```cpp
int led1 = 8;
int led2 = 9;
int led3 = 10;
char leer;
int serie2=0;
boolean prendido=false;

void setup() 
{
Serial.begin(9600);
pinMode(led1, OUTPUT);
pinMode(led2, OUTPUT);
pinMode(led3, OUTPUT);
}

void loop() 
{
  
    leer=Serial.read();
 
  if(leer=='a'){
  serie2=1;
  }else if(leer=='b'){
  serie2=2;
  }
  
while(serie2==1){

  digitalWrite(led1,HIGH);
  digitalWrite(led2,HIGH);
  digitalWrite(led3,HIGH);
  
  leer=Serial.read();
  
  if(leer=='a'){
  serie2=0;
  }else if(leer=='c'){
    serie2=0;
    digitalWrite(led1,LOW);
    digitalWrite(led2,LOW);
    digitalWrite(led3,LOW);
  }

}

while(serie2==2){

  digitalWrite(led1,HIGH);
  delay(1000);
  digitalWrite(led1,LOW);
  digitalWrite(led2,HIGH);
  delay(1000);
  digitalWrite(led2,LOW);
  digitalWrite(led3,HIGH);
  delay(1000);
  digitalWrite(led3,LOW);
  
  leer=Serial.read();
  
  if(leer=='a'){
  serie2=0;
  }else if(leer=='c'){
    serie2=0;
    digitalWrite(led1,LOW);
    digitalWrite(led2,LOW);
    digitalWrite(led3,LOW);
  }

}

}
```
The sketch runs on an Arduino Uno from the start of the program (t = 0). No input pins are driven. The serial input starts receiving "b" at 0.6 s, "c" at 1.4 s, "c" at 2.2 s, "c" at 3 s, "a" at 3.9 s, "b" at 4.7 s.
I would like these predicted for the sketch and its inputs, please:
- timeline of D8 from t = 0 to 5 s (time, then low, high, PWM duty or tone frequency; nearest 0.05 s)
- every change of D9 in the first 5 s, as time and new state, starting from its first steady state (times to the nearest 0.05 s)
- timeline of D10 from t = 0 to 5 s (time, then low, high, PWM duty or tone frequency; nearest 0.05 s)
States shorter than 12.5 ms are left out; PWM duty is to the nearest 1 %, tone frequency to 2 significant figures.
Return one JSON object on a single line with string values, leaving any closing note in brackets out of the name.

{"timeline of D8 from t = 0 to 5 s": "0 s low; 0.6 s high; 1.6 s low; 3.9 s high", "every change of D9 in the first 5 s, as time and new state, starting from its first steady state": "0 s low; 1.6 s high; 2.6 s low; 3.9 s high", "timeline of D10 from t = 0 to 5 s": "0 s low; 2.6 s high; 3.6 s low; 3.9 s high"}
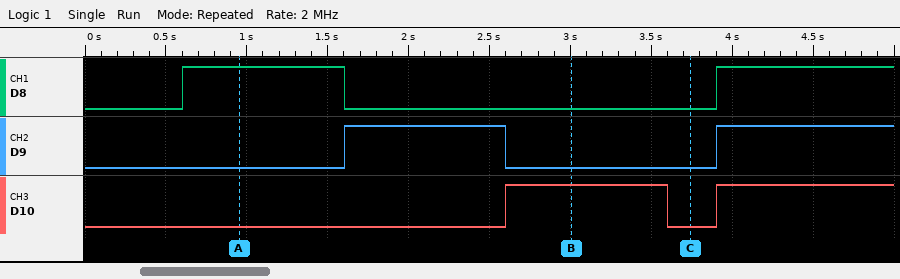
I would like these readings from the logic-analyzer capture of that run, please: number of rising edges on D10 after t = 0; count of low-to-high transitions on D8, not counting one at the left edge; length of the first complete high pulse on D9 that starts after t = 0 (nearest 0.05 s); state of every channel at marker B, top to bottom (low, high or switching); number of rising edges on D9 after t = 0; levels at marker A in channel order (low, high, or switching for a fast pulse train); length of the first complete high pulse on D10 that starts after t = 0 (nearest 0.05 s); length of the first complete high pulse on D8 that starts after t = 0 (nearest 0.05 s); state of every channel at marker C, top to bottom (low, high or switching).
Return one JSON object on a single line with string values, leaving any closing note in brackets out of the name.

{"number of rising edges on D10 after t = 0": "2", "count of low-to-high transitions on D8, not counting one at the left edge": "2", "length of the first complete high pulse on D9 that starts after t = 0": "1.00 s", "state of every channel at marker B, top to bottom": "D8 low, D9 low, D10 high", "number of rising edges on D9 after t = 0": "2", "levels at marker A in channel order": "D8 high, D9 low, D10 low", "length of the first complete high pulse on D10 that starts after t = 0": "1.00 s", "length of the first complete high pulse on D8 that starts after t = 0": "1.00 s", "state of every channel at marker C, top to bottom": "D8 low, D9 low, D10 low"}
